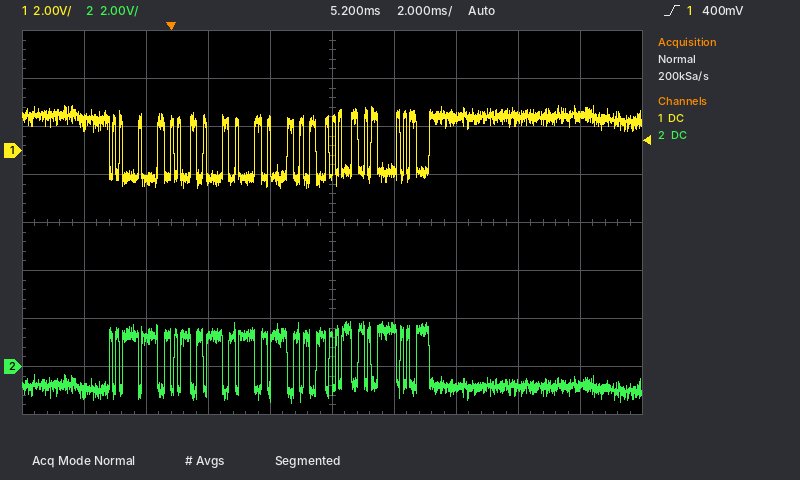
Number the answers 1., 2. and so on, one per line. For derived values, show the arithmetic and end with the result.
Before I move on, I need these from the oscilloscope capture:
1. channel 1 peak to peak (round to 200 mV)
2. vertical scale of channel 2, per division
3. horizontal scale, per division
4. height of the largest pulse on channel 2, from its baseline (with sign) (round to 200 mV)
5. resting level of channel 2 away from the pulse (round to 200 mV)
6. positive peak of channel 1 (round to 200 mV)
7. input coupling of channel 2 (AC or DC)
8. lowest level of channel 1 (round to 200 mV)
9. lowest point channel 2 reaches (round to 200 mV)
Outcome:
1. 1.8 V − (-1.6 V) = 3.4 V
2. 2 V
3. 2 ms
4. +2.8 V
5. -800 mV
6. 1.8 V
7. DC
8. -1.6 V
9. -1.6 V
